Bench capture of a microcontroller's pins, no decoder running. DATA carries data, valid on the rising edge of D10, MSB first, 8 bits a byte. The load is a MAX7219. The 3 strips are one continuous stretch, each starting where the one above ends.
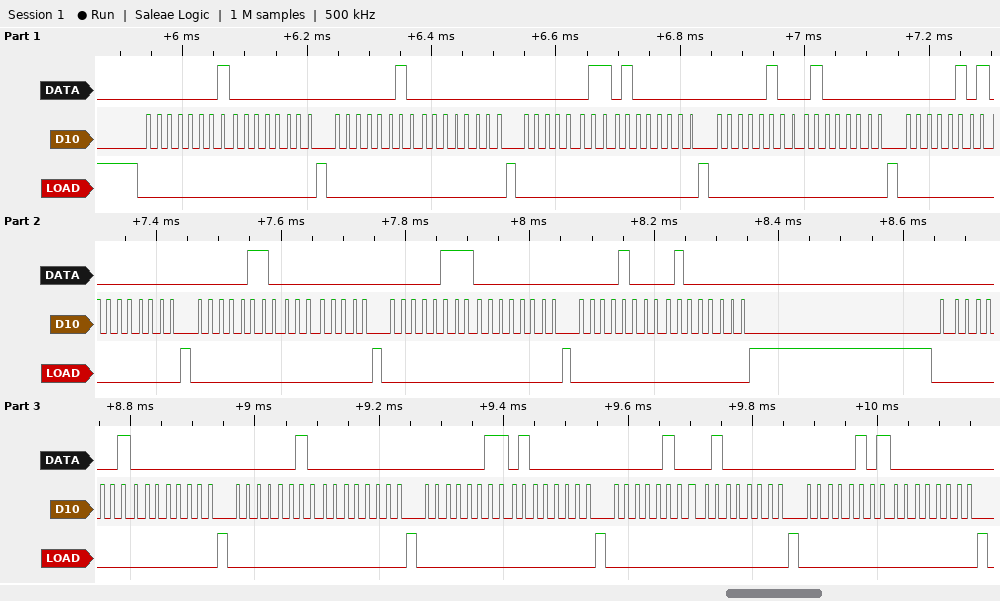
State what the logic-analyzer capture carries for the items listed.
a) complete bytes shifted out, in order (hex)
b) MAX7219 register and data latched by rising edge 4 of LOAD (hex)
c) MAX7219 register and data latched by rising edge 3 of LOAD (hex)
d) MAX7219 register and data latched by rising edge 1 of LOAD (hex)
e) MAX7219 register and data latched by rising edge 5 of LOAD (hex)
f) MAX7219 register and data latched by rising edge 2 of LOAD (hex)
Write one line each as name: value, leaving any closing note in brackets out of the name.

complete bytes shifted out, in order: 01 00 02 00 03 40 04 40 05 00 06 00 07 00 08 40 01 00 02 00 03 40 04 40 05 00
MAX7219 register and data latched by rising edge 4 of LOAD: register 0x4, data 0x40
MAX7219 register and data latched by rising edge 3 of LOAD: register 0x3, data 0x40
MAX7219 register and data latched by rising edge 1 of LOAD: register 0x1, data 0x00
MAX7219 register and data latched by rising edge 5 of LOAD: register 0x5, data 0x00
MAX7219 register and data latched by rising edge 2 of LOAD: register 0x2, data 0x00
